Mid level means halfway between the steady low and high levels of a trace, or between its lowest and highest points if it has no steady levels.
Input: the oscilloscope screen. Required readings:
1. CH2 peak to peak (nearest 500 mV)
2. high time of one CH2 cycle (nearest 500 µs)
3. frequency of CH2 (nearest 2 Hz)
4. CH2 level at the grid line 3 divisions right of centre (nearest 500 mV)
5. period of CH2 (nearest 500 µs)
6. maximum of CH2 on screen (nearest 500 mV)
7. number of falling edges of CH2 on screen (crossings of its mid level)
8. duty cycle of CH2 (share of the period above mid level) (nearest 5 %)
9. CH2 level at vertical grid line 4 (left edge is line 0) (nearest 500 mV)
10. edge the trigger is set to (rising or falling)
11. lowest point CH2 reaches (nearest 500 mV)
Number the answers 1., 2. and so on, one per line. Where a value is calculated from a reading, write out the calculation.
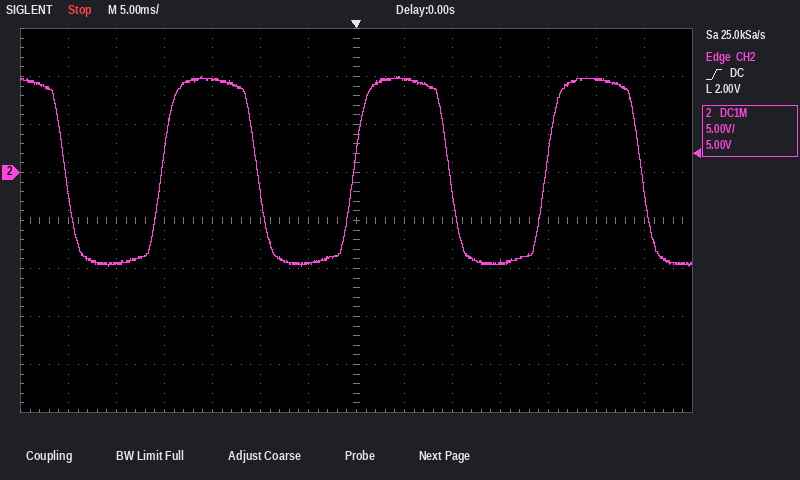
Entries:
1. 10.0 V − (-10.0 V) = 20.0 V
2. 10.0 ms
3. 1 / 20.0 ms ≈ 50 Hz
4. -9.5 V
5. 20.0 ms
6. 10.0 V
7. 4
8. 10.0 ms / 20.0 ms ≈ 50 %
9. 9.5 V
10. rising
11. -10.0 V
